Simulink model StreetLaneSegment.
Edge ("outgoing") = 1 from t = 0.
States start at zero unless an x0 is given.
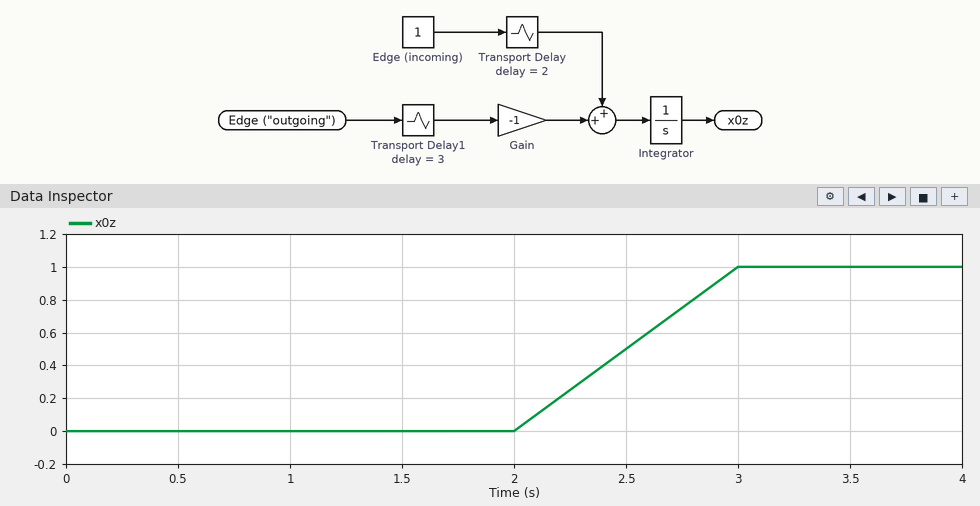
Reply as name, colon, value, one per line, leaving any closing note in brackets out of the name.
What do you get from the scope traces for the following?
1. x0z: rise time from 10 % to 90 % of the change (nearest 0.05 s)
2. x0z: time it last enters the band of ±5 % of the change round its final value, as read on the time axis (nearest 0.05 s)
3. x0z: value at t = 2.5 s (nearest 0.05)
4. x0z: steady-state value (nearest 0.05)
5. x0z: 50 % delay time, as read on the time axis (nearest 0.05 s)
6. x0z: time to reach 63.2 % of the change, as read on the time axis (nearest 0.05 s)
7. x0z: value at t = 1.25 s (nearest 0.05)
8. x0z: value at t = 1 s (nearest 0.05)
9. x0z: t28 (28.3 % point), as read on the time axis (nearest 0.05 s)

x0z: rise time from 10 % to 90 % of the change: 0.80 s
x0z: time it last enters the band of ±5 % of the change round its final value, as read on the time axis: 2.95 s
x0z: value at t = 2.5 s: 0.50
x0z: steady-state value: 1.00
x0z: 50 % delay time, as read on the time axis: 2.50 s
x0z: time to reach 63.2 % of the change, as read on the time axis: 2.65 s
x0z: value at t = 1.25 s: 0.00
x0z: value at t = 1 s: 0.00
x0z: t28 (28.3 % point), as read on the time axis: 2.30 s
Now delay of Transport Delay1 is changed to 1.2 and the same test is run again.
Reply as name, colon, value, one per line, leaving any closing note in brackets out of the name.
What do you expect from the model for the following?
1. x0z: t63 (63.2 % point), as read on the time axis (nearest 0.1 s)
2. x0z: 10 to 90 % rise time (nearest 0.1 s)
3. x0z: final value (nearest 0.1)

x0z: t63 (63.2 % point), as read on the time axis: 1.7 s
x0z: 10 to 90 % rise time: 0.6 s
x0z: final value: -0.8
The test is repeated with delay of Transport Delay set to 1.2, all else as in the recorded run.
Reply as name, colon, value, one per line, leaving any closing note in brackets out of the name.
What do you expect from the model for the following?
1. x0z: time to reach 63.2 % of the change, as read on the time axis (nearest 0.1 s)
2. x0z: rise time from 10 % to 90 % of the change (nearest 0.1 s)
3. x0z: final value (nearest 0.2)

x0z: time to reach 63.2 % of the change, as read on the time axis: 2.3 s
x0z: rise time from 10 % to 90 % of the change: 1.4 s
x0z: final value: 1.8
